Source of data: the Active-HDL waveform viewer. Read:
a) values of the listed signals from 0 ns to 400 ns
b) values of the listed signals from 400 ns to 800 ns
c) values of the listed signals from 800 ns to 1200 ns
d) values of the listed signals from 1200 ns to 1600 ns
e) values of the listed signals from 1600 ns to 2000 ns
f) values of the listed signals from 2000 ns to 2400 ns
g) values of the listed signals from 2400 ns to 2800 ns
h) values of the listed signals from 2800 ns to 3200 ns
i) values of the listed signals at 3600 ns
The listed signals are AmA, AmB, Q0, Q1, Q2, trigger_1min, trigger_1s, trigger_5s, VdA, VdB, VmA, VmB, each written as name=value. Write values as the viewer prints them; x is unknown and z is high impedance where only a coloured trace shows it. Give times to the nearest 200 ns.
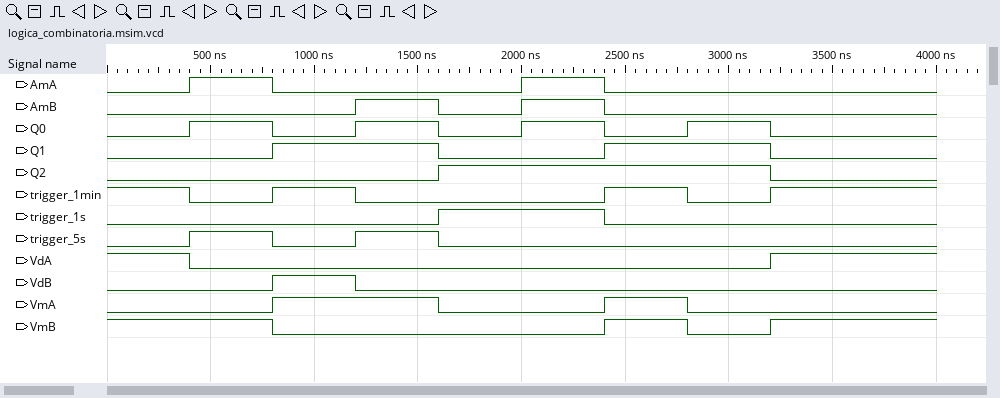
AmA=0, AmB=0, Q0=0, Q1=0, Q2=0, trigger_1min=1, trigger_1s=0, trigger_5s=0, VdA=1, VdB=0, VmA=0, VmB=1
AmA=1, AmB=0, Q0=1, Q1=0, Q2=0, trigger_1min=0, trigger_1s=0, trigger_5s=1, VdA=0, VdB=0, VmA=0, VmB=1
AmA=0, AmB=0, Q0=0, Q1=1, Q2=0, trigger_1min=1, trigger_1s=0, trigger_5s=0, VdA=0, VdB=1, VmA=1, VmB=0
AmA=0, AmB=1, Q0=1, Q1=1, Q2=0, trigger_1min=0, trigger_1s=0, trigger_5s=1, VdA=0, VdB=0, VmA=1, VmB=0
AmA=0, AmB=0, Q0=0, Q1=0, Q2=1, trigger_1min=0, trigger_1s=1, trigger_5s=0, VdA=0, VdB=0, VmA=0, VmB=0
AmA=1, AmB=1, Q0=1, Q1=0, Q2=1, trigger_1min=0, trigger_1s=1, trigger_5s=0, VdA=0, VdB=0, VmA=0, VmB=0
AmA=0, AmB=0, Q0=0, Q1=1, Q2=1, trigger_1min=1, trigger_1s=0, trigger_5s=0, VdA=0, VdB=0, VmA=1, VmB=1
AmA=0, AmB=0, Q0=1, Q1=1, Q2=1, trigger_1min=0, trigger_1s=0, trigger_5s=0, VdA=0, VdB=0, VmA=0, VmB=0
AmA=0, AmB=0, Q0=0, Q1=0, Q2=0, trigger_1min=1, trigger_1s=0, trigger_5s=0, VdA=1, VdB=0, VmA=0, VmB=1
